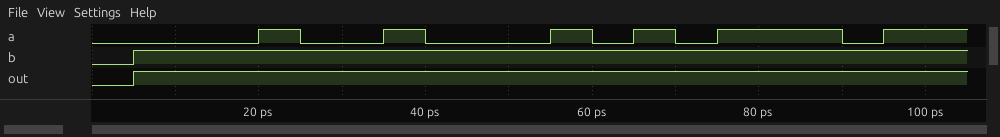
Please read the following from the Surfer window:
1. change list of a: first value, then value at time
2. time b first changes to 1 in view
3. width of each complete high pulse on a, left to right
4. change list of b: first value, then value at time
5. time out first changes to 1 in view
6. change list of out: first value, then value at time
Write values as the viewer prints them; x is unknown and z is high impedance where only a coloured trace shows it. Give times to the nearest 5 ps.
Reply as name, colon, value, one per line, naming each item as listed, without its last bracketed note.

change list of a: first value, then value at time: 0, 1 at 20 ps, 0 at 25 ps, 1 at 35 ps, 0 at 40 ps, 1 at 55 ps, 0 at 60 ps, 1 at 65 ps, 0 at 70 ps, 1 at 75 ps, 0 at 90 ps, 1 at 95 ps
time b first changes to 1 in view: 5 ps
width of each complete high pulse on a, left to right: 5 ps, 5 ps, 5 ps, 5 ps, 15 ps
change list of b: first value, then value at time: 0, 1 at 5 ps
time out first changes to 1 in view: 5 ps
change list of out: first value, then value at time: 0, 1 at 5 ps
